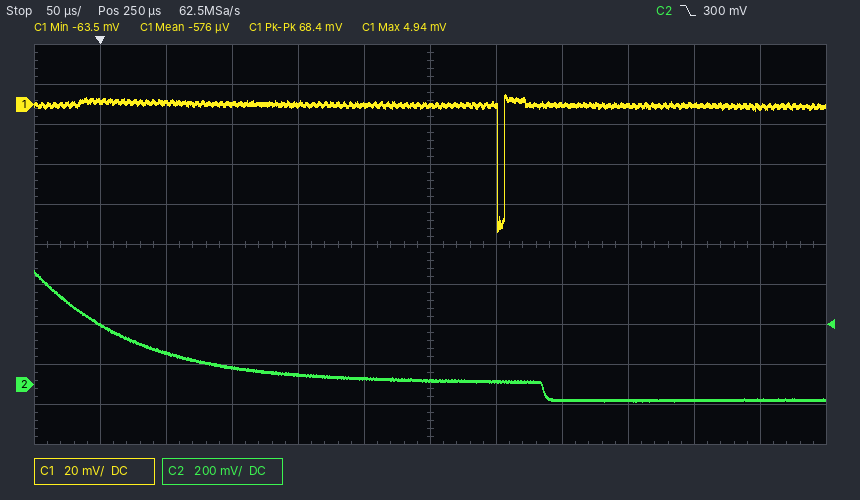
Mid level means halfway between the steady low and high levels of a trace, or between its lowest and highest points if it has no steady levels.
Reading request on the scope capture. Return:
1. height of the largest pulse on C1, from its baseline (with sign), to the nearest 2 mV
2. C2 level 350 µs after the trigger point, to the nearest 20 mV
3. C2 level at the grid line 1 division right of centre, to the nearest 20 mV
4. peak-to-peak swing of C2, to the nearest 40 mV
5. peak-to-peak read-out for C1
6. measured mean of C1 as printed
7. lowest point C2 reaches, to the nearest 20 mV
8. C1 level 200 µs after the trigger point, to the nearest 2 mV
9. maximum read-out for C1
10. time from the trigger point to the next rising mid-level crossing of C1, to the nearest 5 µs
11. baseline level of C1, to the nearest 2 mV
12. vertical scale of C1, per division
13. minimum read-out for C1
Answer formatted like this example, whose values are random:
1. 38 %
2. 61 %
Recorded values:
1. -64 mV
2. -80 mV
3. 20 mV
4. 640 mV
5. 68.4 mV
6. -576 µV
7. -80 mV
8. 0 mV
9. 4.94 mV
10. 305 µs
11. 0 mV
12. 20 mV
13. -63.5 mV
